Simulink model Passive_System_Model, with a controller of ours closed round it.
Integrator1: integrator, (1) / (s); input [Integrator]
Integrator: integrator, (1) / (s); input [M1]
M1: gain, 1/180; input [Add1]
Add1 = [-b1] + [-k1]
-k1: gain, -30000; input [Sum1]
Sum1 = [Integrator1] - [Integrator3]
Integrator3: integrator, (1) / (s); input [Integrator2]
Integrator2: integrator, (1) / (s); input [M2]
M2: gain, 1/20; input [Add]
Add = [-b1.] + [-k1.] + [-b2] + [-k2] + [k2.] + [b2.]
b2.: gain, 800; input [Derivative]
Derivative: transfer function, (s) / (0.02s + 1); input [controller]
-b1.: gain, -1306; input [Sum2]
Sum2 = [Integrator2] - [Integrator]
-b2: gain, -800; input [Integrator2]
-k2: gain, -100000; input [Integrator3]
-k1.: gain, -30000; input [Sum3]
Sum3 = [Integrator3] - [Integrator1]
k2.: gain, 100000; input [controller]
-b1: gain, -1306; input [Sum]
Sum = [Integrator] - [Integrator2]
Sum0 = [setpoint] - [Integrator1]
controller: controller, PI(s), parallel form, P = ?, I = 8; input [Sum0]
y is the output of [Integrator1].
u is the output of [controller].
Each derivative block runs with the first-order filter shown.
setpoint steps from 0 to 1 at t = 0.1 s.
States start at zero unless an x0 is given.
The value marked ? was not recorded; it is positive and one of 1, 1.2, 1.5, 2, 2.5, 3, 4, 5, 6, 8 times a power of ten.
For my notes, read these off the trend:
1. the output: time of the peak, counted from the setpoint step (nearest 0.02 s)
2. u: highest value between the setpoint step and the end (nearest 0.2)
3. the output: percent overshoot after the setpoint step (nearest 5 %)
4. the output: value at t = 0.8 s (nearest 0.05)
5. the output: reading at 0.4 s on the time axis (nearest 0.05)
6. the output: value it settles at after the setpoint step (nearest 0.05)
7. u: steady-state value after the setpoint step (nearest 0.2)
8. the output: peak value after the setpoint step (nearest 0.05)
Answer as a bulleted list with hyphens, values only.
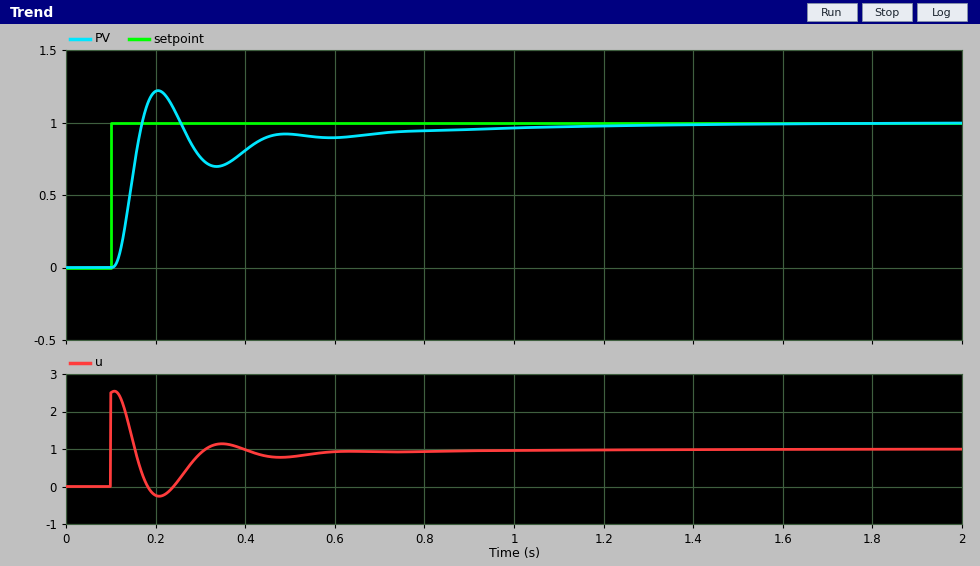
- 0.10 s
- 2.6
- 20 %
- 0.95
- 0.80
- 1.00
- 1.0
- 1.20
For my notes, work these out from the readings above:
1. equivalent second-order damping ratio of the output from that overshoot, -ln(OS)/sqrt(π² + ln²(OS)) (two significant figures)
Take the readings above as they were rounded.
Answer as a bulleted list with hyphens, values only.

- 0.46
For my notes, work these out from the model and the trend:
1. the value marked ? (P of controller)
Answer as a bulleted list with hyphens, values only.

- 2.5
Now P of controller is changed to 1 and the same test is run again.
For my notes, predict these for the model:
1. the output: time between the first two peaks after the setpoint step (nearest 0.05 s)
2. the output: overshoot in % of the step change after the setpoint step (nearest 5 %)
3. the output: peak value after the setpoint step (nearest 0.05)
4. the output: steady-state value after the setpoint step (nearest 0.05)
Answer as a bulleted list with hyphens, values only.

- 0.35 s
- 15 %
- 1.15
- 1.00
